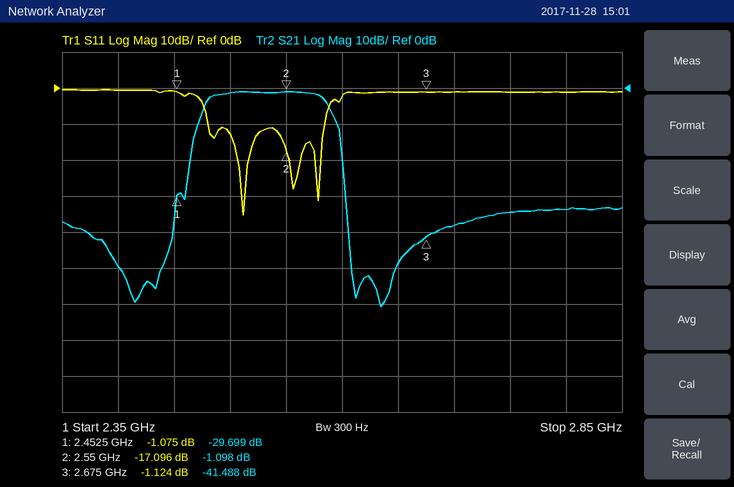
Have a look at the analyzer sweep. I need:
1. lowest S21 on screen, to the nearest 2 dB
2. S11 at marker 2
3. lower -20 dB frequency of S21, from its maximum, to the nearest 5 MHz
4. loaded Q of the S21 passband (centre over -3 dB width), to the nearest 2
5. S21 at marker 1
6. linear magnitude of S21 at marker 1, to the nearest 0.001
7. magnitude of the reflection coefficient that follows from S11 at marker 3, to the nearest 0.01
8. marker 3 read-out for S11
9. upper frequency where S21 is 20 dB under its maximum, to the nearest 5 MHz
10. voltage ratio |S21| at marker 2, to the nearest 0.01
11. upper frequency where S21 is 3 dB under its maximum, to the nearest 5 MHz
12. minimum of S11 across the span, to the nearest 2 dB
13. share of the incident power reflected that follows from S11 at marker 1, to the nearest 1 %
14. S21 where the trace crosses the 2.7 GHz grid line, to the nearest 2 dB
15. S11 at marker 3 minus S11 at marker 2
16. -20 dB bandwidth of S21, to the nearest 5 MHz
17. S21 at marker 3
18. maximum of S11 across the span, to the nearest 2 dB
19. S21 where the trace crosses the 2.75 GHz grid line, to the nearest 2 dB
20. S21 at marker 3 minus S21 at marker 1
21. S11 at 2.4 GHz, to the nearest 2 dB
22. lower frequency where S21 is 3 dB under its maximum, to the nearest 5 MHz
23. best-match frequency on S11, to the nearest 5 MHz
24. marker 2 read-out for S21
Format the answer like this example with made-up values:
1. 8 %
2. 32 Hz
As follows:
1. -60 dB
2. -17.096 dB
3. 2.465 GHz
4. 24
5. -29.699 dB
6. 0.033
7. 0.88
8. -1.124 dB
9. 2.600 GHz
10. 0.88
11. 2.585 GHz
12. -36 dB
13. 78 %
14. -38 dB
15. 15.972 dB
16. 135 MHz
17. -41.488 dB
18. 0 dB
19. -34 dB
20. -11.789 dB
21. 0 dB
22. 2.480 GHz
23. 2.510 GHz
24. -1.098 dB
